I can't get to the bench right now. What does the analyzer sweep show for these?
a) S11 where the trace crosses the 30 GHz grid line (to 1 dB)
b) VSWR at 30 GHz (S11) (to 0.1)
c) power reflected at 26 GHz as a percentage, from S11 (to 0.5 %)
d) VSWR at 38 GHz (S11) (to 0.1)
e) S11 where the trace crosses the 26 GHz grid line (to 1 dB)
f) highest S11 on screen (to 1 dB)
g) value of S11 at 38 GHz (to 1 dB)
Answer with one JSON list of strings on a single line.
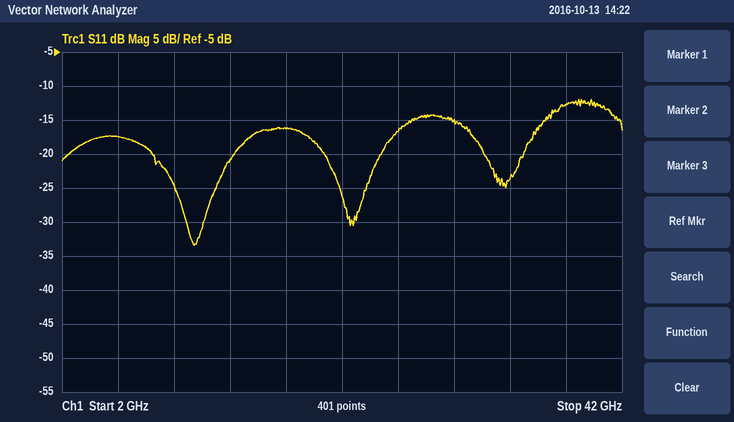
["-15 dB", "1.4", "2.0 %", "1.6", "-17 dB", "-12 dB", "-13 dB"]
